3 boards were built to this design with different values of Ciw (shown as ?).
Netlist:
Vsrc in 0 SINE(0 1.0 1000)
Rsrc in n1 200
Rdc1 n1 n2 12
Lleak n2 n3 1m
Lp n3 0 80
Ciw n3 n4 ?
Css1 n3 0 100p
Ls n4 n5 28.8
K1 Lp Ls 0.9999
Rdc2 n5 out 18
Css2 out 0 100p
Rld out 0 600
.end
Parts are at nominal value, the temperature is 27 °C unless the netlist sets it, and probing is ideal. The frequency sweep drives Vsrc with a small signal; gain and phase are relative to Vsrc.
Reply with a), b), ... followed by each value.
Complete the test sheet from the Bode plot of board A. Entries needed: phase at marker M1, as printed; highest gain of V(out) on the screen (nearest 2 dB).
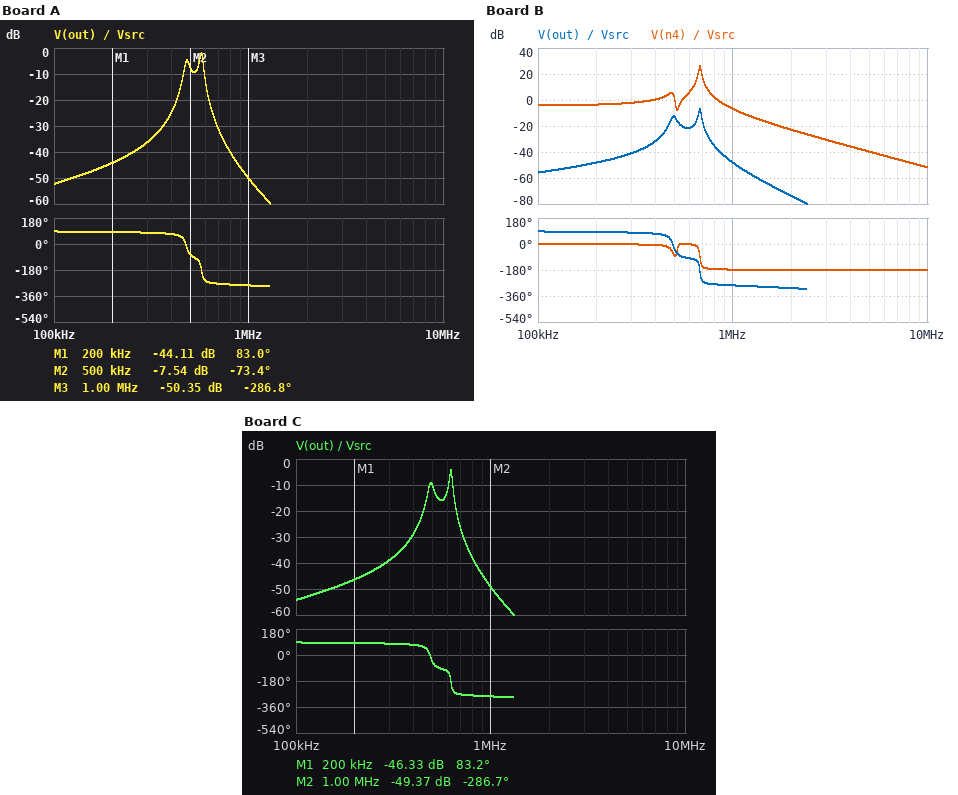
a) 83.0 deg
b) -2 dB
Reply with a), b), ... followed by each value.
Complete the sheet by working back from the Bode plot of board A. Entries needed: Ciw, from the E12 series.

a) 15 pF
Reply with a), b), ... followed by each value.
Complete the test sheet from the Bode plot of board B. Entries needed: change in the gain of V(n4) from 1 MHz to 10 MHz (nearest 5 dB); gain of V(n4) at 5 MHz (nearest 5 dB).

a) -45 dB
b) -40 dB
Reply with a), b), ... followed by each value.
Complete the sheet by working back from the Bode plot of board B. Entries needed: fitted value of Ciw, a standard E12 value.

a) 10 pF
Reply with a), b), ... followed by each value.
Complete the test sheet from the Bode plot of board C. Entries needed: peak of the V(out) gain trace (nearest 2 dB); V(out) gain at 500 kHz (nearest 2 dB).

a) -4 dB
b) -10 dB
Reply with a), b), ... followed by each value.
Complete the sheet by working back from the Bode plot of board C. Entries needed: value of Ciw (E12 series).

a) 12 pF
